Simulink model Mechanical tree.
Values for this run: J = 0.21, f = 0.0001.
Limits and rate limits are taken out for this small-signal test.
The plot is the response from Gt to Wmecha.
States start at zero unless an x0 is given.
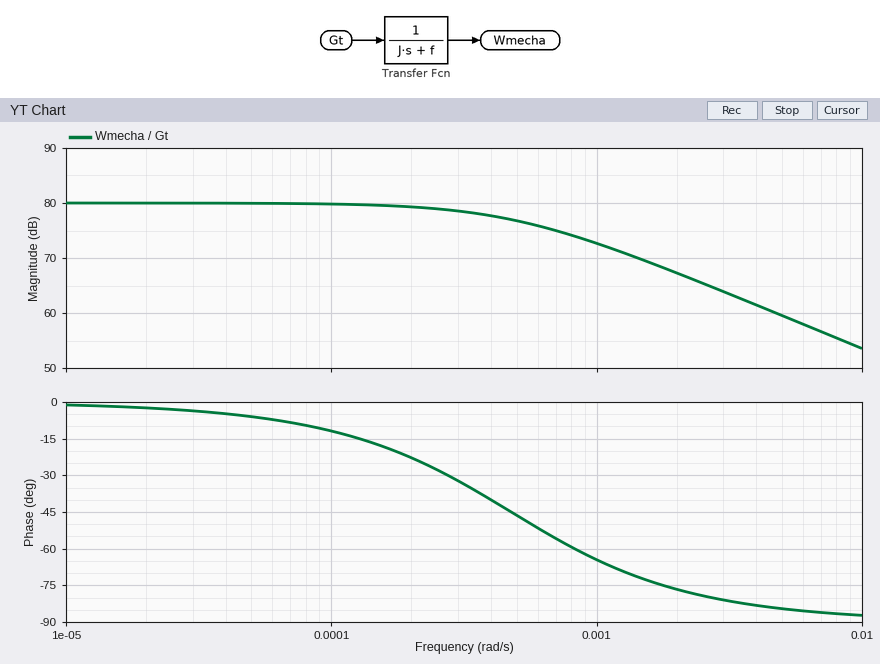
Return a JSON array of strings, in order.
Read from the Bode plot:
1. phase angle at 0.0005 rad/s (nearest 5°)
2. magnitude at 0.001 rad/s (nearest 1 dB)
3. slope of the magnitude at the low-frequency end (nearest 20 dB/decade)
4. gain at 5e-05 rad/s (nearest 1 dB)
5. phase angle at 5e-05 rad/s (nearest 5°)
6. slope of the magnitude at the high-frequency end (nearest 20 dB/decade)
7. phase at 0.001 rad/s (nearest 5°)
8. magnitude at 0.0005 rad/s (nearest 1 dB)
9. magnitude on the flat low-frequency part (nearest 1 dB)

["-45°", "73 dB", "0 dB/decade", "80 dB", "-5°", "-20 dB/decade", "-65°", "77 dB", "80 dB"]
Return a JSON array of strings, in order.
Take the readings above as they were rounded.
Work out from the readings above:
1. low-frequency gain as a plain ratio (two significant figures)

["10000"]
